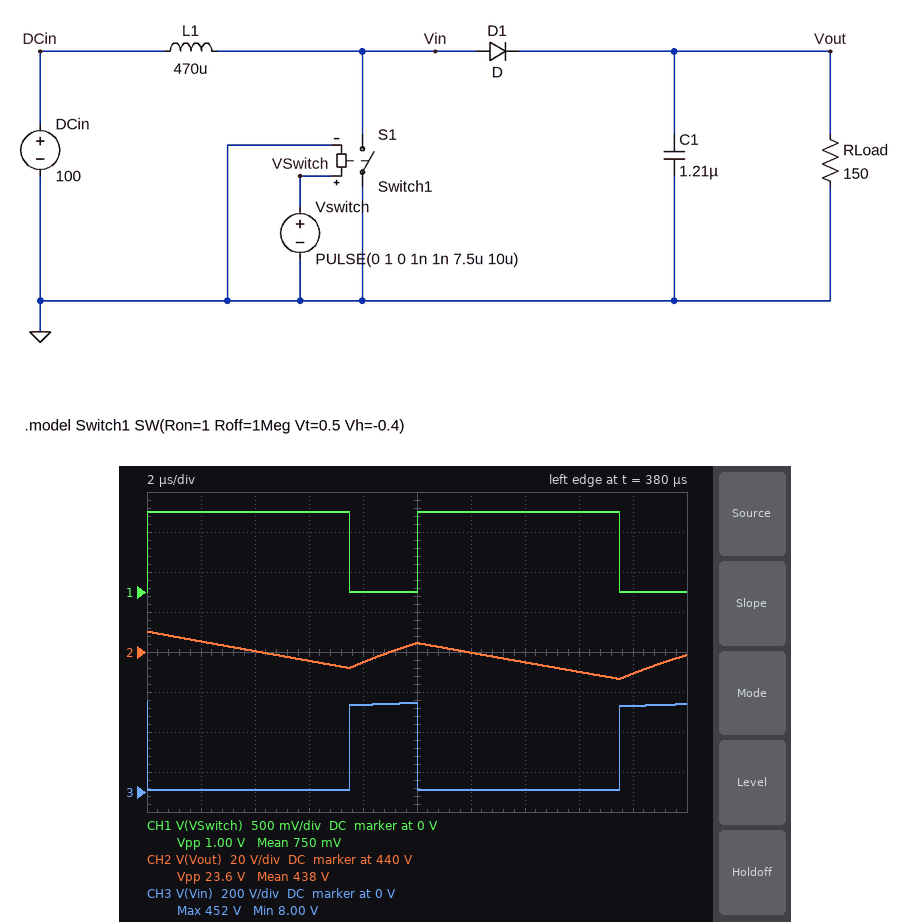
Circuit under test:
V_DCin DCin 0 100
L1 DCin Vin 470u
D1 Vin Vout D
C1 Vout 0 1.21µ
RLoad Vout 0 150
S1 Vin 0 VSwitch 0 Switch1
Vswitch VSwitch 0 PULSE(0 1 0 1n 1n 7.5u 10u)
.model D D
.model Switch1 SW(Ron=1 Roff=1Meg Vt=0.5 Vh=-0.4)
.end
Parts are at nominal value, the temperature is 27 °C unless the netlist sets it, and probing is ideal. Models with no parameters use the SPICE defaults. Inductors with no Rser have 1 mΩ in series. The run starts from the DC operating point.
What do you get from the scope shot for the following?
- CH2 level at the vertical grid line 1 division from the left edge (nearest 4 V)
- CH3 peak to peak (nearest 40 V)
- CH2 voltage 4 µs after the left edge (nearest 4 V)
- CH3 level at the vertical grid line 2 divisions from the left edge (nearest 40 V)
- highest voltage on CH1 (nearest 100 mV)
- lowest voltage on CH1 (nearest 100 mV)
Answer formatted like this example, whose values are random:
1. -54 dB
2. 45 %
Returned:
1. 444 V
2. 440 V
3. 440 V
4. 0 V
5. 1.0 V
6. 0 V
